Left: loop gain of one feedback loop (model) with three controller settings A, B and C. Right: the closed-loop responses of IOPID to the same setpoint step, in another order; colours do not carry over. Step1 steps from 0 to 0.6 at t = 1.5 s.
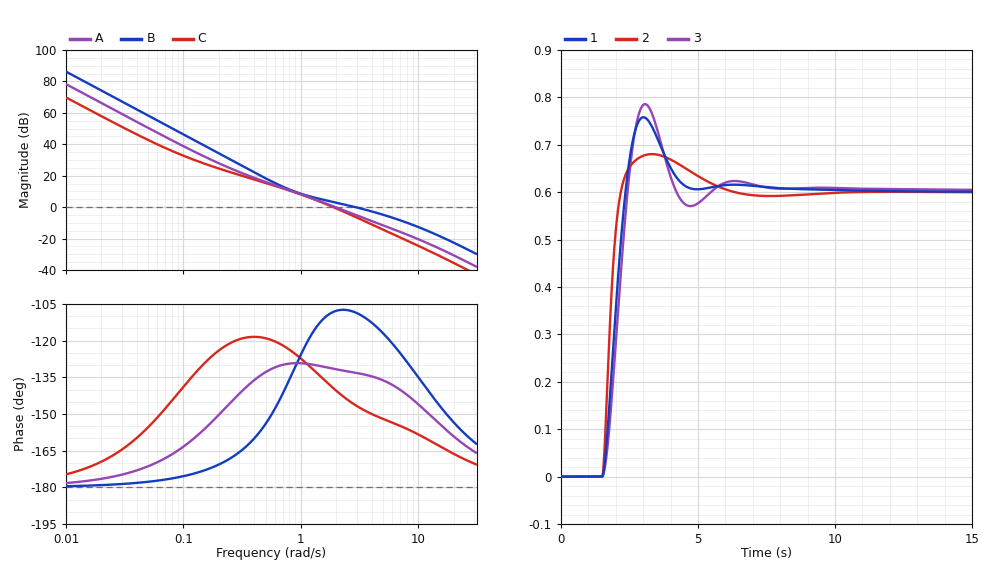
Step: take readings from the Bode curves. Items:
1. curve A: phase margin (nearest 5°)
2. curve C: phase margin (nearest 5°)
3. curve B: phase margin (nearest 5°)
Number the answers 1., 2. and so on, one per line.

1. 50°
2. 40°
3. 70°
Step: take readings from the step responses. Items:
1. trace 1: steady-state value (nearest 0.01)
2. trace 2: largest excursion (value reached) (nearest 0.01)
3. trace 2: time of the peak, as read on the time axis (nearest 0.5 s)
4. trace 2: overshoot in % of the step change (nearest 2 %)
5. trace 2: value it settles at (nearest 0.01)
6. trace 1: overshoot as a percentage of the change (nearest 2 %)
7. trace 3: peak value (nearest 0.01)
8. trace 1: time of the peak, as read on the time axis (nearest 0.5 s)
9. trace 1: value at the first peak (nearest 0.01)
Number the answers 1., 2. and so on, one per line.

1. 0.60
2. 0.68
3. 3.5 s
4. 14 %
5. 0.60
6. 26 %
7. 0.79
8. 3.0 s
9. 0.76
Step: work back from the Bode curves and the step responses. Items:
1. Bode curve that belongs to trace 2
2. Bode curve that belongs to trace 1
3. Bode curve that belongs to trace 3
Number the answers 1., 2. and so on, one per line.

1. B
2. A
3. C
